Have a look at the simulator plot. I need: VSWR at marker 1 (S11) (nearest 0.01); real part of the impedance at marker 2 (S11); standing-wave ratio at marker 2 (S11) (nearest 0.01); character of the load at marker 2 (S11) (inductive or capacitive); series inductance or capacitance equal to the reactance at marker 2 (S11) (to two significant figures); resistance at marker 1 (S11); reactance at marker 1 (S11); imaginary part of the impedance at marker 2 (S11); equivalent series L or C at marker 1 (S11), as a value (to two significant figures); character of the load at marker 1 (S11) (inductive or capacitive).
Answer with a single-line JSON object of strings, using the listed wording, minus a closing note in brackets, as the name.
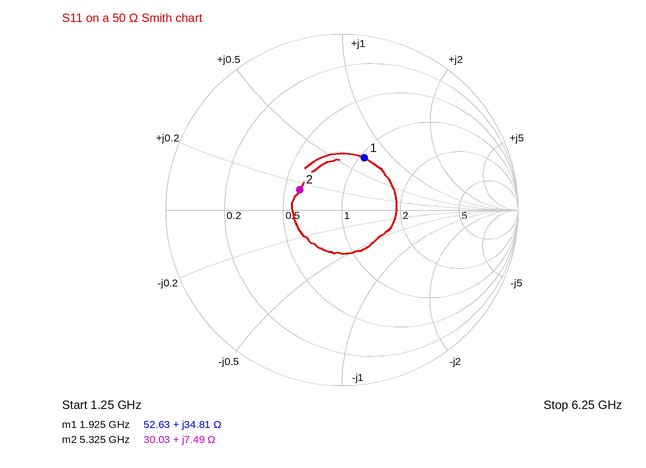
{"VSWR at marker 1 (S11)": "1.95", "real part of the impedance at marker 2": "30.03 Ω", "standing-wave ratio at marker 2 (S11)": "1.72", "character of the load at marker 2 (S11)": "inductive", "series inductance or capacitance equal to the reactance at marker 2 (S11)": "220 pH", "resistance at marker 1": "52.63 Ω", "reactance at marker 1": "+34.81 Ω", "imaginary part of the impedance at marker 2": "+7.49 Ω", "equivalent series L or C at marker 1 (S11), as a value": "2.9 nH", "character of the load at marker 1 (S11)": "inductive"}
